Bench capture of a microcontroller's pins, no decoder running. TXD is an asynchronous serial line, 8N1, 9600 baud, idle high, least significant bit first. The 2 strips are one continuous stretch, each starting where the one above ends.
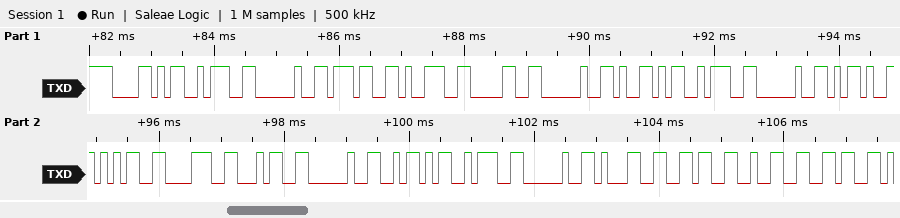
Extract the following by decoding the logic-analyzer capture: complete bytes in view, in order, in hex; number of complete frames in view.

58 3A 20 37 39 30 20 59 3A 20 2D 35 38 34 20 5A 3A 20 31 36 32 36
22
